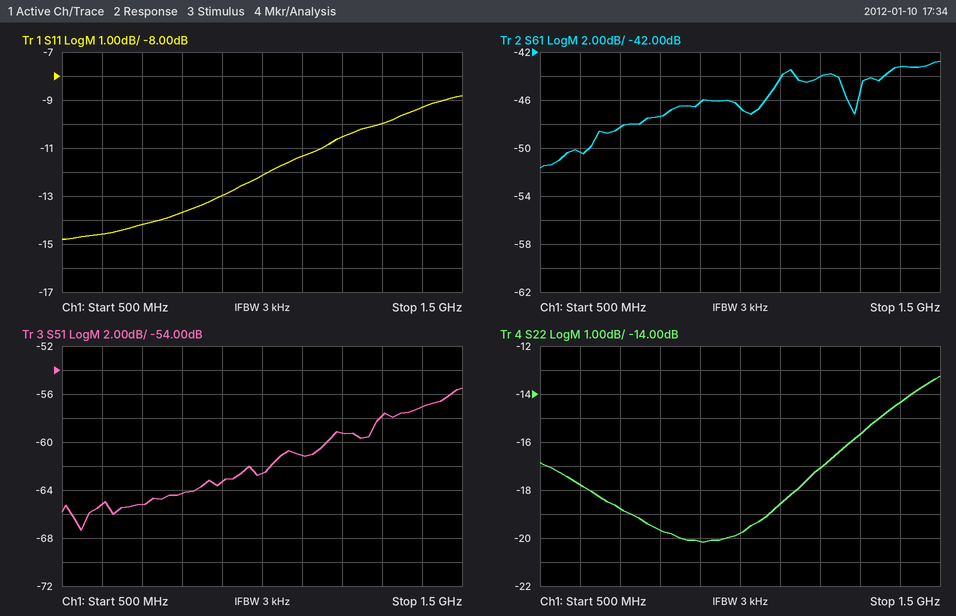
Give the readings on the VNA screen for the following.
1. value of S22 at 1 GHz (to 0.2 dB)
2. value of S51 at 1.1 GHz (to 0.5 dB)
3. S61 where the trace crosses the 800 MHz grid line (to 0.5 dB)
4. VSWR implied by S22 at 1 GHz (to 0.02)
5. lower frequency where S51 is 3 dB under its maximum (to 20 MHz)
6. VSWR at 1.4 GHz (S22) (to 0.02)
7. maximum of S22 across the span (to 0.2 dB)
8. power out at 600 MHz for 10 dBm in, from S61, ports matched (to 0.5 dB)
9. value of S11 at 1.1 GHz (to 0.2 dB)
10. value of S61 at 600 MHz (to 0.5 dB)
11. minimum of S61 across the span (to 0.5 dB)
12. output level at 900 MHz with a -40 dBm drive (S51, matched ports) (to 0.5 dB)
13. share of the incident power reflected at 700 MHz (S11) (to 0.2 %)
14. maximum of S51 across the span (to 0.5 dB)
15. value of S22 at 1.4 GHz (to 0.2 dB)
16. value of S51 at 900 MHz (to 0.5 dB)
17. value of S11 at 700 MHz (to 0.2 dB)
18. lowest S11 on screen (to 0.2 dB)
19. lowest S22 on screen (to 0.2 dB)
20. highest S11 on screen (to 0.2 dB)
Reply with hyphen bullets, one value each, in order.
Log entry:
- -19.8 dB
- -61.0 dB
- -47.5 dB
- 1.22
- 1.28 GHz
- 1.48
- -13.2 dB
- -40.5 dBm
- -11.4 dB
- -50.5 dB
- -51.5 dB
- -103.5 dBm
- 3.8 %
- -55.5 dB
- -14.4 dB
- -63.5 dB
- -14.2 dB
- -14.8 dB
- -20.2 dB
- -8.8 dB
